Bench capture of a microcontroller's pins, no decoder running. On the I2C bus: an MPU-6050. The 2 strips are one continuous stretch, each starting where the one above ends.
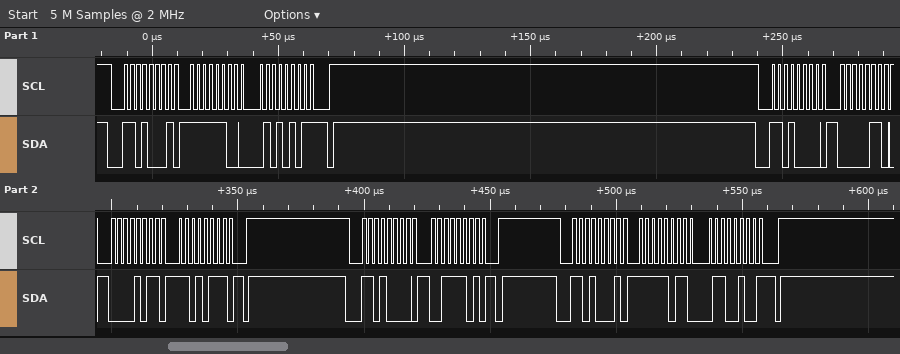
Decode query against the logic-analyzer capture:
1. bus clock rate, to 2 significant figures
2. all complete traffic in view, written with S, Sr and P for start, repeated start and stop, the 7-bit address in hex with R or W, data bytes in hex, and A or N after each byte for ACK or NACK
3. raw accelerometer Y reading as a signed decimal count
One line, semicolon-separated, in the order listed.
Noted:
400 kHz; S 68R A FC A 55 N P S 68W A 06 A 0B A D7 A P S 68W A 3D A P S 68R A FB A 64 N P; -1180
